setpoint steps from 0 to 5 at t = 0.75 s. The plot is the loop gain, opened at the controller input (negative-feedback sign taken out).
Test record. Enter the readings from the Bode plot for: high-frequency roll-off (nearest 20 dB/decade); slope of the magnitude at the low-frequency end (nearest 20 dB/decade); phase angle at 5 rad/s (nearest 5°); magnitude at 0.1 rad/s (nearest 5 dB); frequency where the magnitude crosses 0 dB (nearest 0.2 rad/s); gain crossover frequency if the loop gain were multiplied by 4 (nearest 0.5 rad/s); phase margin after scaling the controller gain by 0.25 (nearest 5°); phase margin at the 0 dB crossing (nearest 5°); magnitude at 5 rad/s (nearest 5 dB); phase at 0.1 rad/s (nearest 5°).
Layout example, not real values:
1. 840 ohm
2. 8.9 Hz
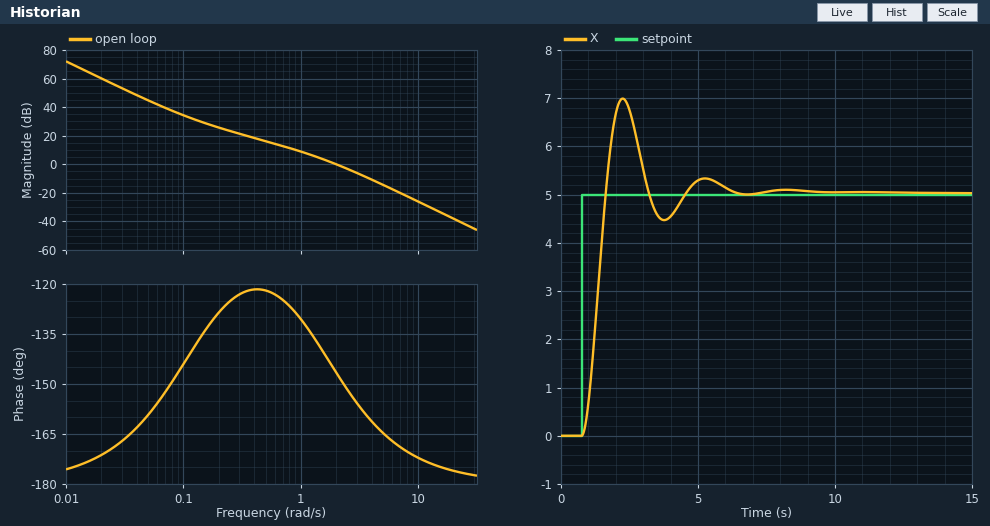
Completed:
1. -40 dB/decade
2. -40 dB/decade
3. -165°
4. 35 dB
5. 2.0 rad/s
6. 4.5 rad/s
7. 55°
8. 35°
9. -15 dB
10. -145°
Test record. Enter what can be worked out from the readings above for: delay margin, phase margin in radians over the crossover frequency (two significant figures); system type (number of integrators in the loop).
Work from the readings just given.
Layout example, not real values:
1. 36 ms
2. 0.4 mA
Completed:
1. 0.31 s
2. 2
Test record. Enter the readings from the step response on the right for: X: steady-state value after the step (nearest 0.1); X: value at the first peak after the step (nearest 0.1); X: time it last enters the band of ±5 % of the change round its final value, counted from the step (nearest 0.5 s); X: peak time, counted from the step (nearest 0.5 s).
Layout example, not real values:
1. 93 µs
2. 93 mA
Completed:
1. 5.0
2. 7.0
3. 5.0 s
4. 1.5 s
